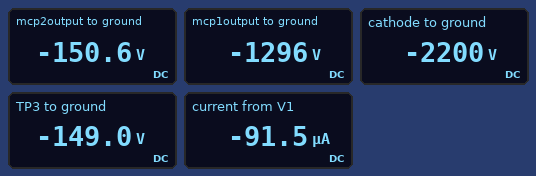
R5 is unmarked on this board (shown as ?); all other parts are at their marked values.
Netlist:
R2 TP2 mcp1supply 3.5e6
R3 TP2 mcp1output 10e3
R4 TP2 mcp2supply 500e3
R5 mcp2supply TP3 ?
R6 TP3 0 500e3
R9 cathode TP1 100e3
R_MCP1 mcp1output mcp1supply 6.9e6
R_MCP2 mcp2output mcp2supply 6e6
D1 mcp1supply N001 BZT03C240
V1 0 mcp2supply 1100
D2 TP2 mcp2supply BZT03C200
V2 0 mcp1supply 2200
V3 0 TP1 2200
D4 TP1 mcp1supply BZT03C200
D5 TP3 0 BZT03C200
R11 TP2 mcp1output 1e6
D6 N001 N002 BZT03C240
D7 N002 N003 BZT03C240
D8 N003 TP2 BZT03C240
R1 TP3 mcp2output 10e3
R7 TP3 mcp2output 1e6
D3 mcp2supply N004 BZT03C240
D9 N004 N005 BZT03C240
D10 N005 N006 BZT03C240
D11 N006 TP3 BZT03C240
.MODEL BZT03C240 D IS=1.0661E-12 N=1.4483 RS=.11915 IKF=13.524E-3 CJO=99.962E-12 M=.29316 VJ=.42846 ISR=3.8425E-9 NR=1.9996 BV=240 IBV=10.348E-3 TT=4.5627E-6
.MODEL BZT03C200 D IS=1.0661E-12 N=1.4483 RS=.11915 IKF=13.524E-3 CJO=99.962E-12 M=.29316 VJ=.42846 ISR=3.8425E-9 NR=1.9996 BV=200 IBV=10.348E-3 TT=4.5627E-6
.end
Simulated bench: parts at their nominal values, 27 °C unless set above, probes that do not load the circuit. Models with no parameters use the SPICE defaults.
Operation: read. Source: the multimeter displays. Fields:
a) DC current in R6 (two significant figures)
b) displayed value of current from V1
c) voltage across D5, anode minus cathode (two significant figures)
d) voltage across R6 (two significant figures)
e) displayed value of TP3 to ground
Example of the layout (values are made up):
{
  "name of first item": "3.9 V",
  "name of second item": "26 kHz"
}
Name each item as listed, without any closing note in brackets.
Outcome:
{
  "DC current in R6": "300 µA",
  "displayed value of current from V1": "-91.5 µA",
  "voltage across D5, anode minus cathode": "-150 V",
  "voltage across R6": "150 V",
  "displayed value of TP3 to ground": "-149.0 V"
}
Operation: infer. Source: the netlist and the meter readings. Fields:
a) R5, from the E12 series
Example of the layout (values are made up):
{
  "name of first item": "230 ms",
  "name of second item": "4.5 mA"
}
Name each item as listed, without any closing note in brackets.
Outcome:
{
  "R5, from the E12 series": "6.8 MΩ"
}
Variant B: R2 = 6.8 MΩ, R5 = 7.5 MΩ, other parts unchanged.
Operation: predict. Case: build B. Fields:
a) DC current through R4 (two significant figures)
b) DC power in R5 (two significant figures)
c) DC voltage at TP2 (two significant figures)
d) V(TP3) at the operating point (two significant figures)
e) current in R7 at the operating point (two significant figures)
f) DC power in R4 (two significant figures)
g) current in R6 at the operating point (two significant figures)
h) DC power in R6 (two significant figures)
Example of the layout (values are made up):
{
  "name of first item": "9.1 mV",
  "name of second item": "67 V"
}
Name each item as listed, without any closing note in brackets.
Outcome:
{
  "DC current through R4": "280 µA",
  "DC power in R5": "120 mW",
  "DC voltage at TP2": "-1.2 kV",
  "V(TP3) at the operating point": "-140 V",
  "current in R7 at the operating point": "1.6 µA",
  "DC power in R4": "40 mW",
  "current in R6 at the operating point": "290 µA",
  "DC power in R6": "41 mW"
}
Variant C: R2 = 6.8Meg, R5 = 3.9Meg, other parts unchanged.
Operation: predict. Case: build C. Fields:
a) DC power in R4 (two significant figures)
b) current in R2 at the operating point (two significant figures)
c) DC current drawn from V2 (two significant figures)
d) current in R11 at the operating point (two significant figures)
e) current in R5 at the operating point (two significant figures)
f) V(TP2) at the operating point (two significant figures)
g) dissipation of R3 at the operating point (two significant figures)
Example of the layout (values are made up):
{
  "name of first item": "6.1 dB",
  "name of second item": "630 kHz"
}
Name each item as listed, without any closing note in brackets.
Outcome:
{
  "DC power in R4": "40 mW",
  "current in R2 at the operating point": "140 µA",
  "DC current drawn from V2": "280 µA",
  "current in R11 at the operating point": "1.4 µA",
  "current in R5 at the operating point": "230 µA",
  "V(TP2) at the operating point": "-1.2 kV",
  "dissipation of R3 at the operating point": "190 µW"
}
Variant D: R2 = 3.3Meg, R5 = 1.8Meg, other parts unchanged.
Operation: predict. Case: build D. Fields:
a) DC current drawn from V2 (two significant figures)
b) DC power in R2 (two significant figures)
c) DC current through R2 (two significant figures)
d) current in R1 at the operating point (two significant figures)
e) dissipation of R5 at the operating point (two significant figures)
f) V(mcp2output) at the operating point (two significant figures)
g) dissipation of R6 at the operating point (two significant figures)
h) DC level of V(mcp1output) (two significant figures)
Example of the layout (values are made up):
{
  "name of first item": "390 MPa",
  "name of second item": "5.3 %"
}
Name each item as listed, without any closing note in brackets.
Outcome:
{
  "DC current drawn from V2": "400 µA",
  "DC power in R2": "250 mW",
  "DC current through R2": "270 µA",
  "current in R1 at the operating point": "150 µA",
  "dissipation of R5 at the operating point": "450 mW",
  "V(mcp2output) at the operating point": "-200 V",
  "dissipation of R6 at the operating point": "80 mW",
  "DC level of V(mcp1output)": "-1.3 kV"
}
